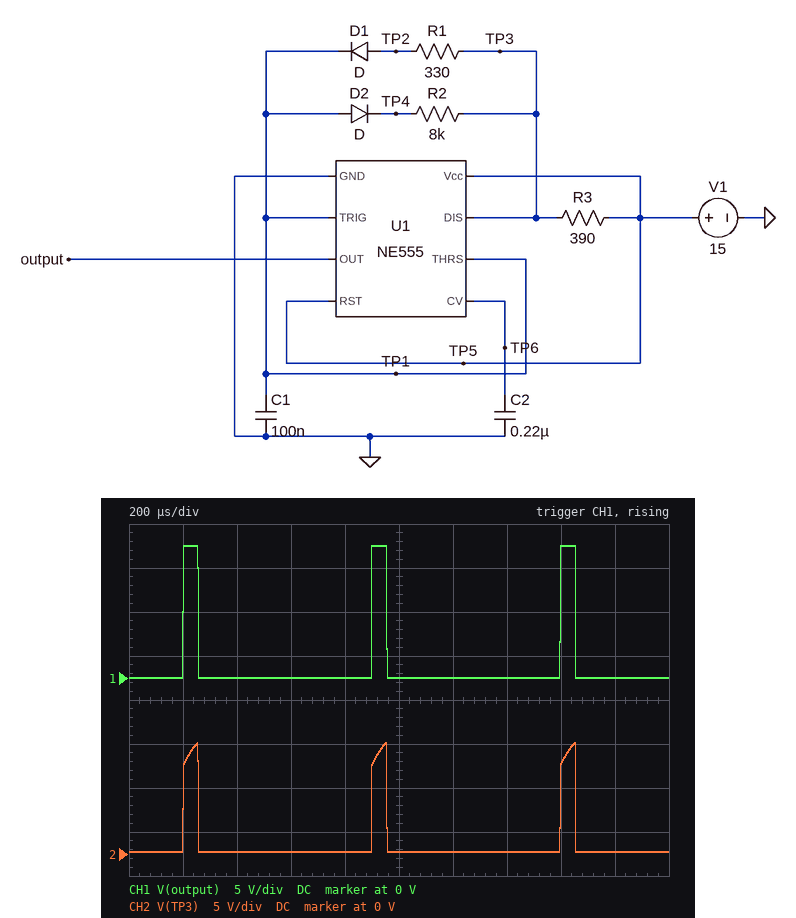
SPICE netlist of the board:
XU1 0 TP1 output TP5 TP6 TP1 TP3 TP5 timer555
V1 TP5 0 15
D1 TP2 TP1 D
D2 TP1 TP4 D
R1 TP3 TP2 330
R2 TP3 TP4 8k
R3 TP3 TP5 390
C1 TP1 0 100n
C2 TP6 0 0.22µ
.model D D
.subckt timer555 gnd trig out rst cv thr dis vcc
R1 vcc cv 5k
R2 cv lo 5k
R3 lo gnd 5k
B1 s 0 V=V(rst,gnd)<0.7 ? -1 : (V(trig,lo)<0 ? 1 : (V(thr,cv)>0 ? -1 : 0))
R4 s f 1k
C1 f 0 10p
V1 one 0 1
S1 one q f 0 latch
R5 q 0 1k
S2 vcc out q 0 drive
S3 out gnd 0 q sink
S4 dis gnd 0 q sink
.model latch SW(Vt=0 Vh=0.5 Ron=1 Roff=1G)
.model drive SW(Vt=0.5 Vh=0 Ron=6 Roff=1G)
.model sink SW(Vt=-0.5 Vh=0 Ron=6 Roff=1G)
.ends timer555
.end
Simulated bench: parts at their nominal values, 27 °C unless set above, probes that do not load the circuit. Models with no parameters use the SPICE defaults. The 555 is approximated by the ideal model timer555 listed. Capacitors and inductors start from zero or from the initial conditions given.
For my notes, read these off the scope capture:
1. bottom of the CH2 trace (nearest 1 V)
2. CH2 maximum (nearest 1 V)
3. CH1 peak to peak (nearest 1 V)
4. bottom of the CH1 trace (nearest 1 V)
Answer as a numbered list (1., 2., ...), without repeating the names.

1. 0 V
2. 13 V
3. 15 V
4. 0 V
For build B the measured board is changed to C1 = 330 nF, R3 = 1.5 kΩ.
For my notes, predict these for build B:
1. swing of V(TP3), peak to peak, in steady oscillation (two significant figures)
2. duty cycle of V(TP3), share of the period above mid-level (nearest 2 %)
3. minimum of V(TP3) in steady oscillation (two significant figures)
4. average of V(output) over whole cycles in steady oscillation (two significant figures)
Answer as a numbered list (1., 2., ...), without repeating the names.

1. 11 V
2. 18 %
3. 63 mV
4. 2.8 V
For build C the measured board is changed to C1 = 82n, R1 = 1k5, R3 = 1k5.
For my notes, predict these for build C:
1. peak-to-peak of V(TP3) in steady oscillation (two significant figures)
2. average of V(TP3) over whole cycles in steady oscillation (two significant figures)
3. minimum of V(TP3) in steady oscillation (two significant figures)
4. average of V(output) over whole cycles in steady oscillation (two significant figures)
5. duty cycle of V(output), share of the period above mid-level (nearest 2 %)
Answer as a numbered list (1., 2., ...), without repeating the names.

1. 13 V
2. 3.2 V
3. 63 mV
4. 4.1 V
5. 28 %
